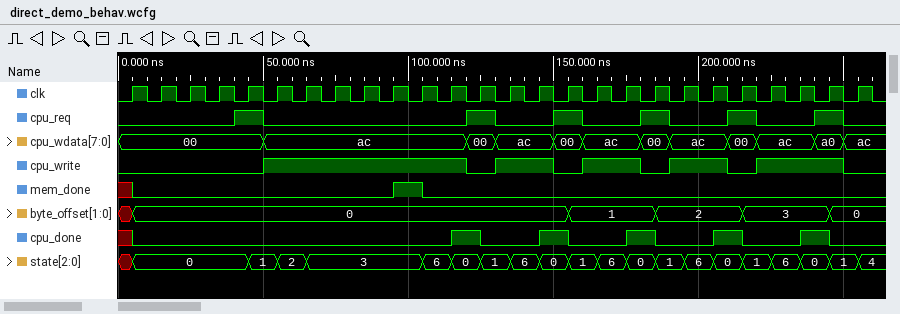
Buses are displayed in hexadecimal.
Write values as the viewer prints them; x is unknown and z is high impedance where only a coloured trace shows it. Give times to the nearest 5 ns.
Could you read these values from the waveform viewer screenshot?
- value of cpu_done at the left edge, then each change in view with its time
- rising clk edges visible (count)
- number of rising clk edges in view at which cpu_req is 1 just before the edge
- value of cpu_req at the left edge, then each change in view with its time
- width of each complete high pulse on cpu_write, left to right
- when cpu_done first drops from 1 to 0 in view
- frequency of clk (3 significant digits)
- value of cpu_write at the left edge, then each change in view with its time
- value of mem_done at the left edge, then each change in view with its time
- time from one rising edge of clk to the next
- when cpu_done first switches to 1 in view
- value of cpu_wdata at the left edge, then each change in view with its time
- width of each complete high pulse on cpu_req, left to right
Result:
x, 0 at 5 ns, 1 at 115 ns, 0 at 125 ns, 1 at 145 ns, 0 at 155 ns, 1 at 175 ns, 0 at 185 ns, 1 at 205 ns, 0 at 215 ns, 1 at 235 ns, 0 at 245 ns
26
6
0, 1 at 40 ns, 0 at 50 ns, 1 at 120 ns, 0 at 130 ns, 1 at 150 ns, 0 at 160 ns, 1 at 180 ns, 0 at 190 ns, 1 at 210 ns, 0 at 220 ns, 1 at 240 ns, 0 at 250 ns
70 ns, 20 ns, 20 ns, 20 ns, 30 ns
125 ns
100 MHz
0, 1 at 50 ns, 0 at 120 ns, 1 at 130 ns, 0 at 150 ns, 1 at 160 ns, 0 at 180 ns, 1 at 190 ns, 0 at 210 ns, 1 at 220 ns, 0 at 250 ns
x, 0 at 5 ns, 1 at 95 ns, 0 at 105 ns
10 ns
115 ns
00, ac at 50 ns, 00 at 120 ns, ac at 130 ns, 00 at 150 ns, ac at 160 ns, 00 at 180 ns, ac at 190 ns, 00 at 210 ns, ac at 220 ns, a0 at 240 ns, ac at 250 ns
10 ns, 10 ns, 10 ns, 10 ns, 10 ns, 10 ns
